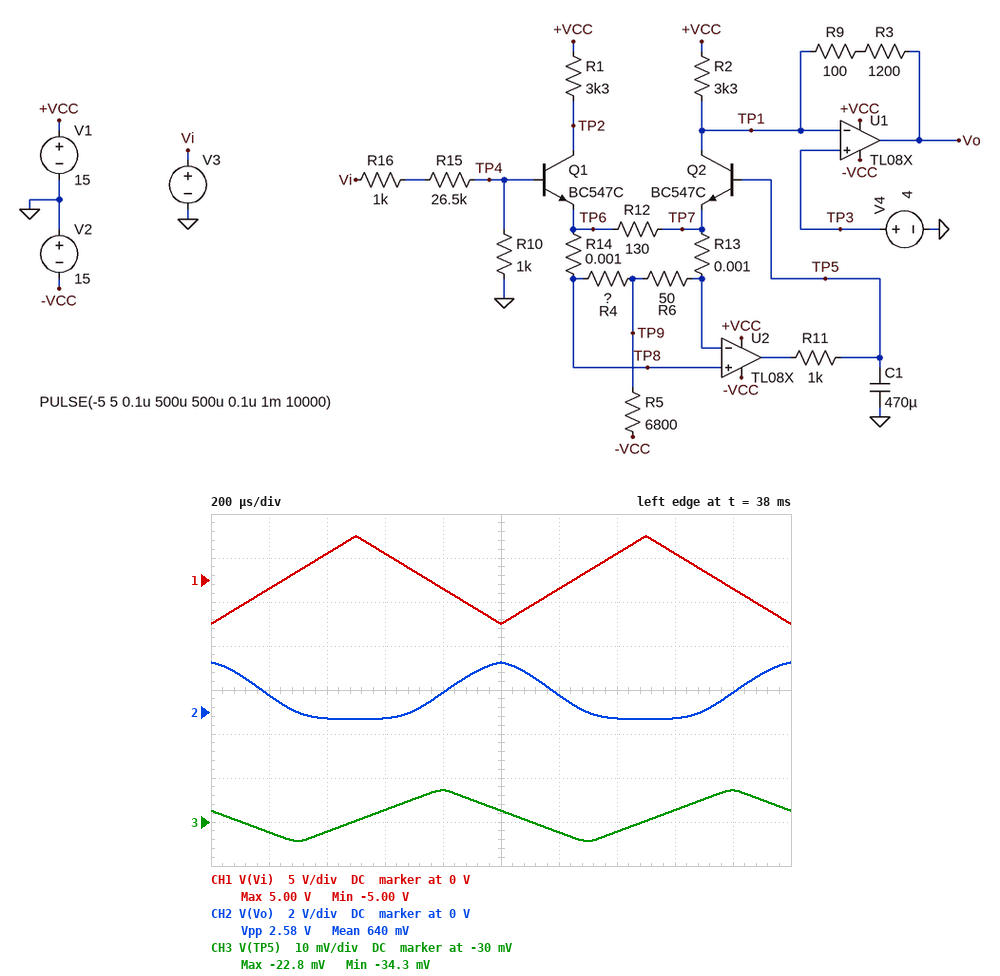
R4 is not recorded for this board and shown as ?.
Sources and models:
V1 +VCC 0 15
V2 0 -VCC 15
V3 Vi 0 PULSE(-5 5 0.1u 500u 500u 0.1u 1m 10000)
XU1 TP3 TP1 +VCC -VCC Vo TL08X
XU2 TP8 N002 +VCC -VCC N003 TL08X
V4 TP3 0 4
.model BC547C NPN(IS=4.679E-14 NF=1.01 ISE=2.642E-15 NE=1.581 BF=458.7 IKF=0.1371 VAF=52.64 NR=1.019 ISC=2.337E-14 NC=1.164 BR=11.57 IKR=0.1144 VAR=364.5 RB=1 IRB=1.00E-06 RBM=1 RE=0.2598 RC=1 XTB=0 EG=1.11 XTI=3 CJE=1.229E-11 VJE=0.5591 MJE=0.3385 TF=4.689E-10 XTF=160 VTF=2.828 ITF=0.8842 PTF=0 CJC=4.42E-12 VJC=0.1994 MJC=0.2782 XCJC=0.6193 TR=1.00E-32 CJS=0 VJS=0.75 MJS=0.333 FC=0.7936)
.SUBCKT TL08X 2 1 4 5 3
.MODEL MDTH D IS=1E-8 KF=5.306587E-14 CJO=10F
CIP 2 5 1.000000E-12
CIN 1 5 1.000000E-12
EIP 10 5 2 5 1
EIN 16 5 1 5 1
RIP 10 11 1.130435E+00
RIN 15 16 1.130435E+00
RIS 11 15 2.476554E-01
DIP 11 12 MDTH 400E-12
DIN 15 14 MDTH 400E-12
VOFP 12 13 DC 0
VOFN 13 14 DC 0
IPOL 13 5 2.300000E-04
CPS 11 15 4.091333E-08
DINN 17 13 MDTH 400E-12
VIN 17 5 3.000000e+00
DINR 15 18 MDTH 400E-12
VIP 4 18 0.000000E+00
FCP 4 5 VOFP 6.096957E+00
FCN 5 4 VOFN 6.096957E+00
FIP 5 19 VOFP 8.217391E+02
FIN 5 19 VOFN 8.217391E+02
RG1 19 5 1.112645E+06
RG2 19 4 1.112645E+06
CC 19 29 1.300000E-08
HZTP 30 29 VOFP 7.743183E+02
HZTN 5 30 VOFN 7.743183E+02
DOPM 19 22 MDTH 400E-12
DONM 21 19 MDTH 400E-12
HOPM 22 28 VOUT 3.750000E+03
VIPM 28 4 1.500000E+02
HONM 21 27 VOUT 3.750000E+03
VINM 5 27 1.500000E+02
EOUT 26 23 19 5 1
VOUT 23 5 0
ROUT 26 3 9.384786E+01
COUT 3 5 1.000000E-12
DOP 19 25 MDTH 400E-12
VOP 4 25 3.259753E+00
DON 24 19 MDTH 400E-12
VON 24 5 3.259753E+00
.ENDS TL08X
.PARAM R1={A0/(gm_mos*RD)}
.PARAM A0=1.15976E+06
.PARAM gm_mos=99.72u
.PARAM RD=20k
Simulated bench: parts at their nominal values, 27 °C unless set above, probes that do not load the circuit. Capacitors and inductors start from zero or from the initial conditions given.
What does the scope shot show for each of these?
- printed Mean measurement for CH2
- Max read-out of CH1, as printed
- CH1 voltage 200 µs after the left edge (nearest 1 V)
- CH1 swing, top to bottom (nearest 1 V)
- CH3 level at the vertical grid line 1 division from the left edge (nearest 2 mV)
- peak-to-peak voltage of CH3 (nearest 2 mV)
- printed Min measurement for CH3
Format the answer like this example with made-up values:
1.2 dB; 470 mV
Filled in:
640 mV; 5.00 V; -1 V; 10 V; -32 mV; 12 mV; -34.3 mV
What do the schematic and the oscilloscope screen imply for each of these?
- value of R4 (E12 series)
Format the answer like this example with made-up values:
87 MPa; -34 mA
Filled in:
18 Ω
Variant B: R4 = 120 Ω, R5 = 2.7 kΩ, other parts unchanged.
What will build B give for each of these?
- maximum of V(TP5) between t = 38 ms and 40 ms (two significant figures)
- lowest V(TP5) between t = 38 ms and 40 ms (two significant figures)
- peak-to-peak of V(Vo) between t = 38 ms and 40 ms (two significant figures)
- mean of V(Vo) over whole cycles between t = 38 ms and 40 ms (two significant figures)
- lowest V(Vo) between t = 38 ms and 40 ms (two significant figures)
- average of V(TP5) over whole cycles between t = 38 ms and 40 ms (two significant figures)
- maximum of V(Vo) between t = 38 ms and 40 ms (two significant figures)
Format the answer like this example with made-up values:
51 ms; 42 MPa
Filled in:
29 mV; 17 mV; 4.1 V; 4.4 V; 2.2 V; 23 mV; 6.3 V
